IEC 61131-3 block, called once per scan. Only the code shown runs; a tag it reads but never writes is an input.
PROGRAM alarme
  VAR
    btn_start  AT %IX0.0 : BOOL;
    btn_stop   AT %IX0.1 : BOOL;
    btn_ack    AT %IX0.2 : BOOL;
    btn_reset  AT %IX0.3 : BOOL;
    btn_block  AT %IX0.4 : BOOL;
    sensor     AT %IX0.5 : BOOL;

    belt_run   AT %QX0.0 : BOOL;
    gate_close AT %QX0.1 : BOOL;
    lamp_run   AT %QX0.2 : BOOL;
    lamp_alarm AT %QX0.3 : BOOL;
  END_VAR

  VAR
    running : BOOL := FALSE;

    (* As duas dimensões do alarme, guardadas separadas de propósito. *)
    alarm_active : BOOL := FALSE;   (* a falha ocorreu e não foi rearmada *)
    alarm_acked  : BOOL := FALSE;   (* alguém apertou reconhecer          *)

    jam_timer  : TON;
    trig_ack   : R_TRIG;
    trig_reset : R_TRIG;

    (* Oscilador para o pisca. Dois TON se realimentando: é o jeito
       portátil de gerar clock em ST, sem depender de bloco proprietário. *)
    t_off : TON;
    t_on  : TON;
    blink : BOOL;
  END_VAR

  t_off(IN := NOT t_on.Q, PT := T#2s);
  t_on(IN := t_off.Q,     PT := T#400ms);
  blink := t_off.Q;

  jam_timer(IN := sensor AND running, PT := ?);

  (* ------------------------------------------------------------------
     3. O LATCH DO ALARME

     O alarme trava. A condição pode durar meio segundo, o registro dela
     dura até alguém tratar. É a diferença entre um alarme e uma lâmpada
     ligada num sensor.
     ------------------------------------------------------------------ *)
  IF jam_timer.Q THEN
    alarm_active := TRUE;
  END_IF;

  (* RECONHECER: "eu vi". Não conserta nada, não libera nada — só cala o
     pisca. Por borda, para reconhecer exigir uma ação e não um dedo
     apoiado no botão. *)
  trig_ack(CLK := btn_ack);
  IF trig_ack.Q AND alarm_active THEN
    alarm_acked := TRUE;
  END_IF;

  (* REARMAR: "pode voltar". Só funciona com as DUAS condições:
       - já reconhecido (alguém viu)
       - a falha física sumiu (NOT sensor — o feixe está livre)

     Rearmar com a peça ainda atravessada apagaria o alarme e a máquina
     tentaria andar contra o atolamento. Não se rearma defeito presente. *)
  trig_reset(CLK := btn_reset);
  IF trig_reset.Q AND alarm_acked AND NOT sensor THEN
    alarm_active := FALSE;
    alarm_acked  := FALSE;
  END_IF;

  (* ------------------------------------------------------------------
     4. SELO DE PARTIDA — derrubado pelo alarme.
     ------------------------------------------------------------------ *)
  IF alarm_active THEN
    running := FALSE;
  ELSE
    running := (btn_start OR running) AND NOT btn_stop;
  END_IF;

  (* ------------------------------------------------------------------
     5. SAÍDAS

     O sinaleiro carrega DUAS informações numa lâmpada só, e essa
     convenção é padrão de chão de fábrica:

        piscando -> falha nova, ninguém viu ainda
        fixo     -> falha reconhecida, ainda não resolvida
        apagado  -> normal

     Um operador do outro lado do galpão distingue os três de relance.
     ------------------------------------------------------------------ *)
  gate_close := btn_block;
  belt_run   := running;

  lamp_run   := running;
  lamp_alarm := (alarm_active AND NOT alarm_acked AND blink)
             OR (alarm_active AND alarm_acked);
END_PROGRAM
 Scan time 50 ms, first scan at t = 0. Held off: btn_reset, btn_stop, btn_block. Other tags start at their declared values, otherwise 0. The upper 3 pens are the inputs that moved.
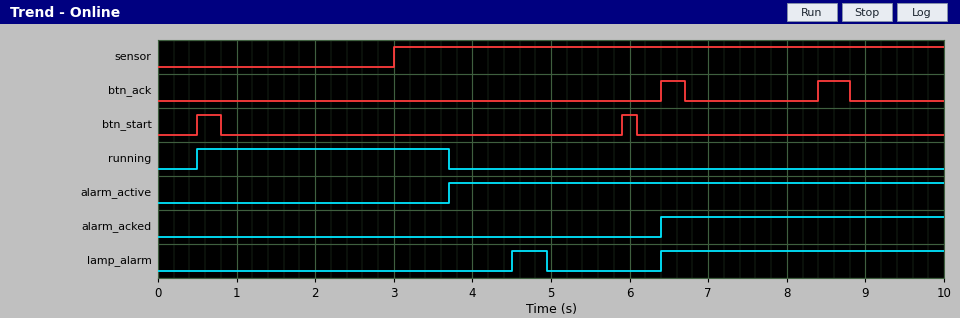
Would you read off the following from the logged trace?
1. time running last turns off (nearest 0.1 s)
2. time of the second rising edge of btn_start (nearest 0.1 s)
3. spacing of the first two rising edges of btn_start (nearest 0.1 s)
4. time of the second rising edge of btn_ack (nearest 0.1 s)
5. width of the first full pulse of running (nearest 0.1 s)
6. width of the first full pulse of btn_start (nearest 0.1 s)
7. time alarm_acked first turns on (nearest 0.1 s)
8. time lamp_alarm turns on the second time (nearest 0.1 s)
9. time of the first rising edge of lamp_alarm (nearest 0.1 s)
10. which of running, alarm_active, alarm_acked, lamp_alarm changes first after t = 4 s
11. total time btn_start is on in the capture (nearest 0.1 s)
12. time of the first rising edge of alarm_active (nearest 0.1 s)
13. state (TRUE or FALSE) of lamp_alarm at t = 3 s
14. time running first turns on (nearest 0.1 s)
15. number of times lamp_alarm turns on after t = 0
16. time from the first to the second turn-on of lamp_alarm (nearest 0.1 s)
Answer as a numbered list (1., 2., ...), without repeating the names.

1. 3.7 s
2. 5.9 s
3. 5.4 s
4. 8.4 s
5. 3.2 s
6. 0.3 s
7. 6.4 s
8. 6.4 s
9. 4.5 s
10. lamp_alarm
11. 0.5 s
12. 3.7 s
13. FALSE
14. 0.5 s
15. 2
16. 1.9 s
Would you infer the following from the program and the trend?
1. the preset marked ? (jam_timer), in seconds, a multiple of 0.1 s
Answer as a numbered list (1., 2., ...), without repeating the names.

1. 0.7 s
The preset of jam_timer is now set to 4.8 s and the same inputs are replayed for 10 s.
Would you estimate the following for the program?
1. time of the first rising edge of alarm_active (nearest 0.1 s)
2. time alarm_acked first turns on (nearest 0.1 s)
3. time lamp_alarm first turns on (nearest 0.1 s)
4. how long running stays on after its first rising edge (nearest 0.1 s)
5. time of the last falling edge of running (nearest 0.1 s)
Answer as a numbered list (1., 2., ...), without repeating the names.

1. 7.8 s
2. 8.4 s
3. 8.4 s
4. 7.3 s
5. 7.8 s
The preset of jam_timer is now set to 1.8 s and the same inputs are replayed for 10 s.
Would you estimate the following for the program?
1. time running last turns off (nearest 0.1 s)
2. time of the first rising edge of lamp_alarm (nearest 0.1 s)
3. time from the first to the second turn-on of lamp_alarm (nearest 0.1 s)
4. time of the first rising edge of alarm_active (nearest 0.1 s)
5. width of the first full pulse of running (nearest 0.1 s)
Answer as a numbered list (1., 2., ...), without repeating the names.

1. 4.8 s
2. 4.8 s
3. 1.6 s
4. 4.8 s
5. 4.3 s
